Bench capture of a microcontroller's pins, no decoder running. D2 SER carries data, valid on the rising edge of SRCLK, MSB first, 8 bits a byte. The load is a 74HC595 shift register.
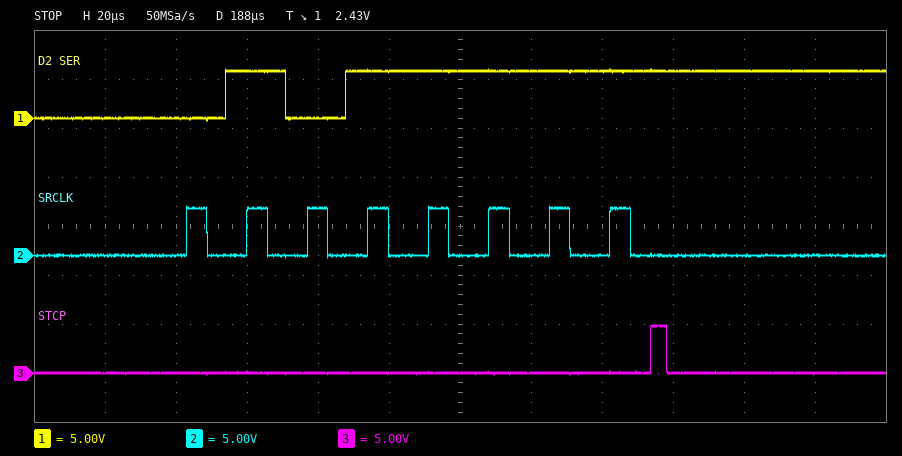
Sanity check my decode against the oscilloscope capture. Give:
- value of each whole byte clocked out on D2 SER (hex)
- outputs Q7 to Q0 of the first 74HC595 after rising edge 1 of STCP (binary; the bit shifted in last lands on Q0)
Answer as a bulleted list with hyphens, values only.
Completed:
- 5F
- 01011111
